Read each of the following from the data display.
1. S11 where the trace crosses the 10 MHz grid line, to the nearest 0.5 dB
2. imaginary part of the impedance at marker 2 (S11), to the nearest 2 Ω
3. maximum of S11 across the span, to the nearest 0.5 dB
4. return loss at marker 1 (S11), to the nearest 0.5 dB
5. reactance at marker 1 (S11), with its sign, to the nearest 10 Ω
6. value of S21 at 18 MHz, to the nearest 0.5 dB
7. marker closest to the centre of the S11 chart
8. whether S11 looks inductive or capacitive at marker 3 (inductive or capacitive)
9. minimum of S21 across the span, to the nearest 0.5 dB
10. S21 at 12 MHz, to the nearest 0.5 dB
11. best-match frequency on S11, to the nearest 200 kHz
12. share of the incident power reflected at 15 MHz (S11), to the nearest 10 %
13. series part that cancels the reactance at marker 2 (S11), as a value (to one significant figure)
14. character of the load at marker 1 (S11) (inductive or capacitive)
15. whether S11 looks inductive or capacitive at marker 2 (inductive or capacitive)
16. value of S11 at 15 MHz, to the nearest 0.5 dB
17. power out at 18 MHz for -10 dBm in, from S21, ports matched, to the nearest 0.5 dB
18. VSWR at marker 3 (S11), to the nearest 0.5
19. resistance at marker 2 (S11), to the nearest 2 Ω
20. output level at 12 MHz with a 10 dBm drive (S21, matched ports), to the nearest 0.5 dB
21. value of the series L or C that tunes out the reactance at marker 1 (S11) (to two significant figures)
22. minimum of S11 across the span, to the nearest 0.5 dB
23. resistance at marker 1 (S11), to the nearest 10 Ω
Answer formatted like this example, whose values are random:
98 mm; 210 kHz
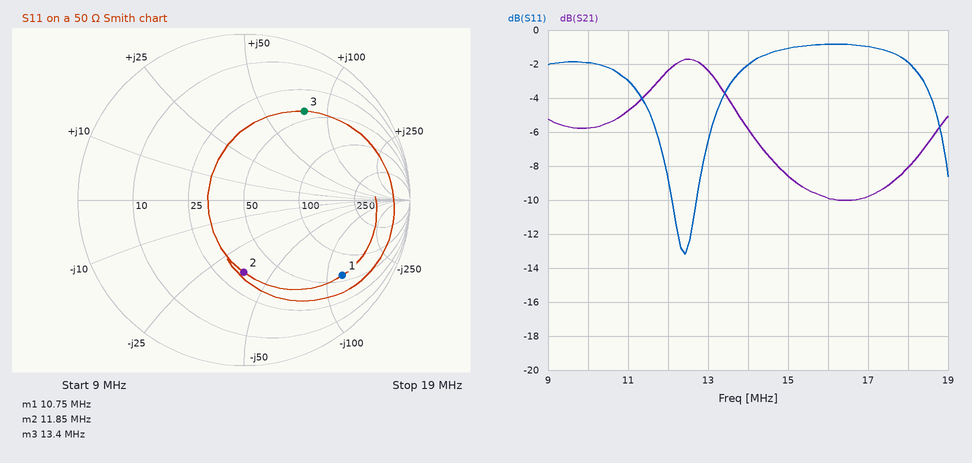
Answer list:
-2.0 dB; -36 Ω; -1.0 dB; 2.5 dB; -120 Ω; -8.0 dB; marker 2; inductive; -10.0 dB; -2.5 dB; 12.4 MHz; 80 %; 500 nH; capacitive; capacitive; -1.0 dB; -18.0 dBm; 4.5; 34 Ω; 7.5 dBm; 1.8 µH; -13.0 dB; 60 Ω
